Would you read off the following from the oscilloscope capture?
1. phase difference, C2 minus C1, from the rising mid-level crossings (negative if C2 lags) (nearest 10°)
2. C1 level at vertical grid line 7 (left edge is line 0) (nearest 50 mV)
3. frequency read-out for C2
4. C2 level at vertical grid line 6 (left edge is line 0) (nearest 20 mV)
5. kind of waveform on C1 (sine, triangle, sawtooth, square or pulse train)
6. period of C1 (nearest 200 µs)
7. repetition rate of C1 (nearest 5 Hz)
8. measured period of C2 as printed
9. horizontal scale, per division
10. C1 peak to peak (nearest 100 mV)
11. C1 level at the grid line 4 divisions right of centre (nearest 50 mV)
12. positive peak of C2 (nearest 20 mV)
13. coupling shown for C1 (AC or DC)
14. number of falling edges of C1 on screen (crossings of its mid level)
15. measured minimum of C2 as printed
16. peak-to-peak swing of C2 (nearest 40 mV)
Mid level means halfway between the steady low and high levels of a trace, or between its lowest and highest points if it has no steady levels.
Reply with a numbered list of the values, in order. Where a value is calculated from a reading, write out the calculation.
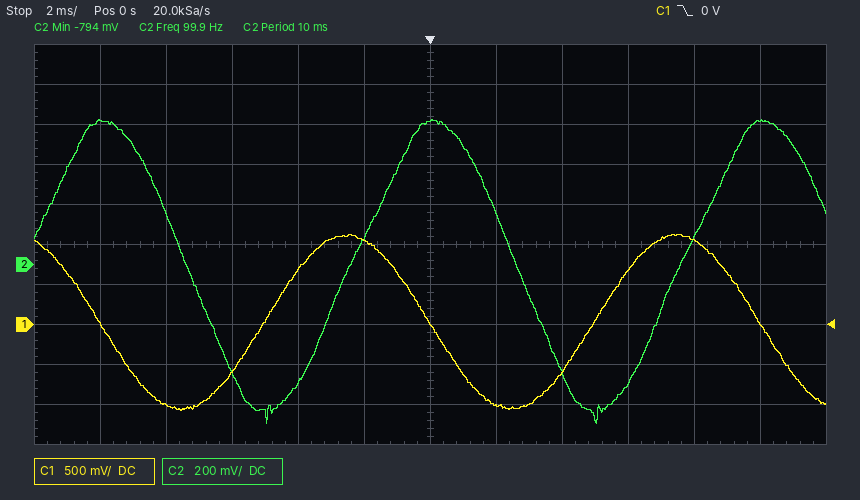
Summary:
1. -90°
2. -1.00 V
3. 99.9 Hz
4. 720 mV
5. sine
6. 10.0 ms
7. 1 / 10.0 ms ≈ 100 Hz
8. 10 ms
9. 2 ms
10. 2.20 V
11. 1.05 V
12. 720 mV
13. DC
14. 3
15. -794 mV
16. 1.52 V
